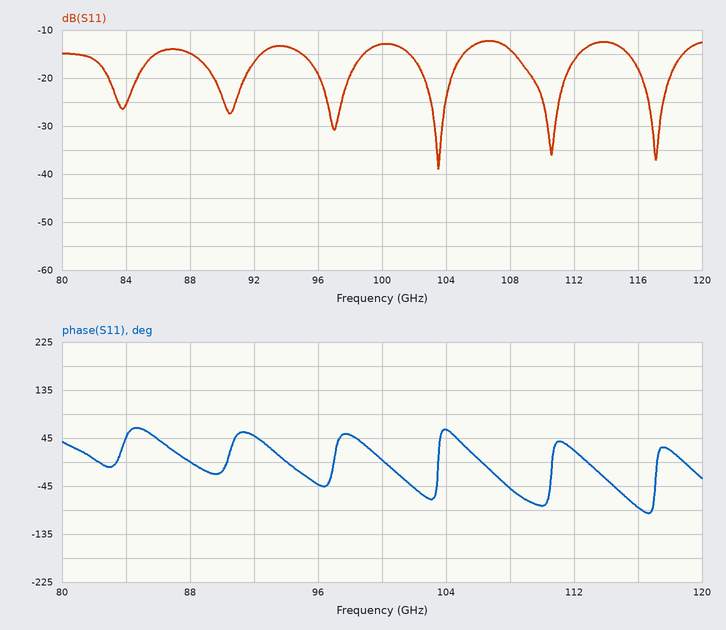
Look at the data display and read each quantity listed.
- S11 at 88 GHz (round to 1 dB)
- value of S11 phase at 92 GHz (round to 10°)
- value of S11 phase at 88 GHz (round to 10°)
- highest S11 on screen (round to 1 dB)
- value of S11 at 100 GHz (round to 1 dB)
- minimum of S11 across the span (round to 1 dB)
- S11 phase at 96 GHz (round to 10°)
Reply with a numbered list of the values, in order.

1. -15 dB
2. 50°
3. 0°
4. -12 dB
5. -13 dB
6. -39 dB
7. -40°
